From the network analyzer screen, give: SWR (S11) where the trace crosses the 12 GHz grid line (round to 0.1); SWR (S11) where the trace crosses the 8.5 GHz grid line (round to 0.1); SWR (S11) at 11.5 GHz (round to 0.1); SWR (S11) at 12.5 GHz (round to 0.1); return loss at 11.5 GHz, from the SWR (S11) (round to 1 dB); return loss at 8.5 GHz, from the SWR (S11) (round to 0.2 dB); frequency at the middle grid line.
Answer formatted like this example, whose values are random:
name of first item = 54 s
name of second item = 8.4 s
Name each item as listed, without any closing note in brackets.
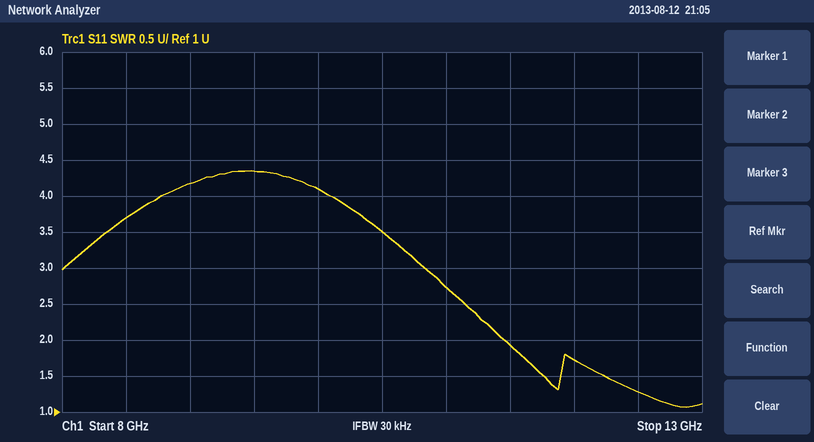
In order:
SWR (S11) where the trace crosses the 12 GHz grid line = 1.7
SWR (S11) where the trace crosses the 8.5 GHz grid line = 3.7
SWR (S11) at 11.5 GHz = 1.9
SWR (S11) at 12.5 GHz = 1.3
return loss at 11.5 GHz, from the SWR (S11) = 10 dB
return loss at 8.5 GHz, from the SWR (S11) = 4.8 dB
frequency at the middle grid line = 10.5 GHz
